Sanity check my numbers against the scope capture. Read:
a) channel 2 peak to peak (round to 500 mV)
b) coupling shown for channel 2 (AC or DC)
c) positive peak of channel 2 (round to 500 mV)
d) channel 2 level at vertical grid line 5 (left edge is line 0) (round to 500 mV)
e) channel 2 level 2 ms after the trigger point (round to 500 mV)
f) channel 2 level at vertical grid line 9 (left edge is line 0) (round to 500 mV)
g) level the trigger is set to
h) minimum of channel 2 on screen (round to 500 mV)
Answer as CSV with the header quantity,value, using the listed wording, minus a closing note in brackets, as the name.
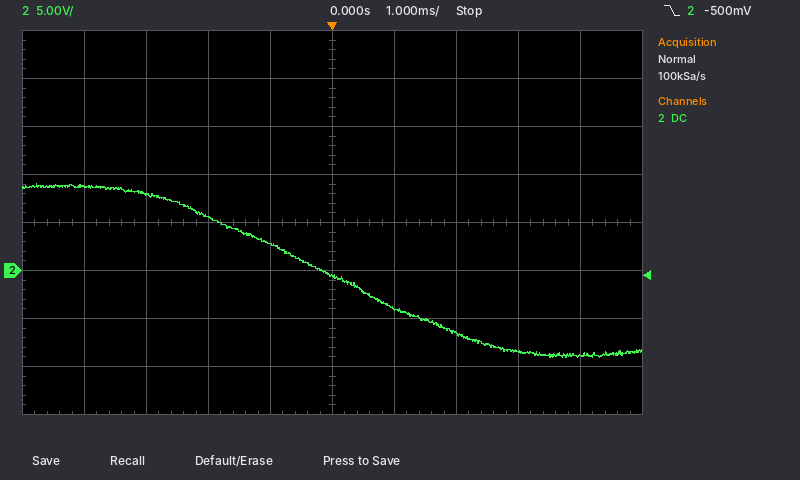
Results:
quantity,value
channel 2 peak to peak,18.0 V
coupling shown for channel 2,DC
positive peak of channel 2,9.0 V
channel 2 level at vertical grid line 5 (left edge is line 0),-500 mV
channel 2 level 2 ms after the trigger point,-6.5 V
channel 2 level at vertical grid line 9 (left edge is line 0),-9.0 V
level the trigger is set to,-500 mV
minimum of channel 2 on screen,-9.0 V
